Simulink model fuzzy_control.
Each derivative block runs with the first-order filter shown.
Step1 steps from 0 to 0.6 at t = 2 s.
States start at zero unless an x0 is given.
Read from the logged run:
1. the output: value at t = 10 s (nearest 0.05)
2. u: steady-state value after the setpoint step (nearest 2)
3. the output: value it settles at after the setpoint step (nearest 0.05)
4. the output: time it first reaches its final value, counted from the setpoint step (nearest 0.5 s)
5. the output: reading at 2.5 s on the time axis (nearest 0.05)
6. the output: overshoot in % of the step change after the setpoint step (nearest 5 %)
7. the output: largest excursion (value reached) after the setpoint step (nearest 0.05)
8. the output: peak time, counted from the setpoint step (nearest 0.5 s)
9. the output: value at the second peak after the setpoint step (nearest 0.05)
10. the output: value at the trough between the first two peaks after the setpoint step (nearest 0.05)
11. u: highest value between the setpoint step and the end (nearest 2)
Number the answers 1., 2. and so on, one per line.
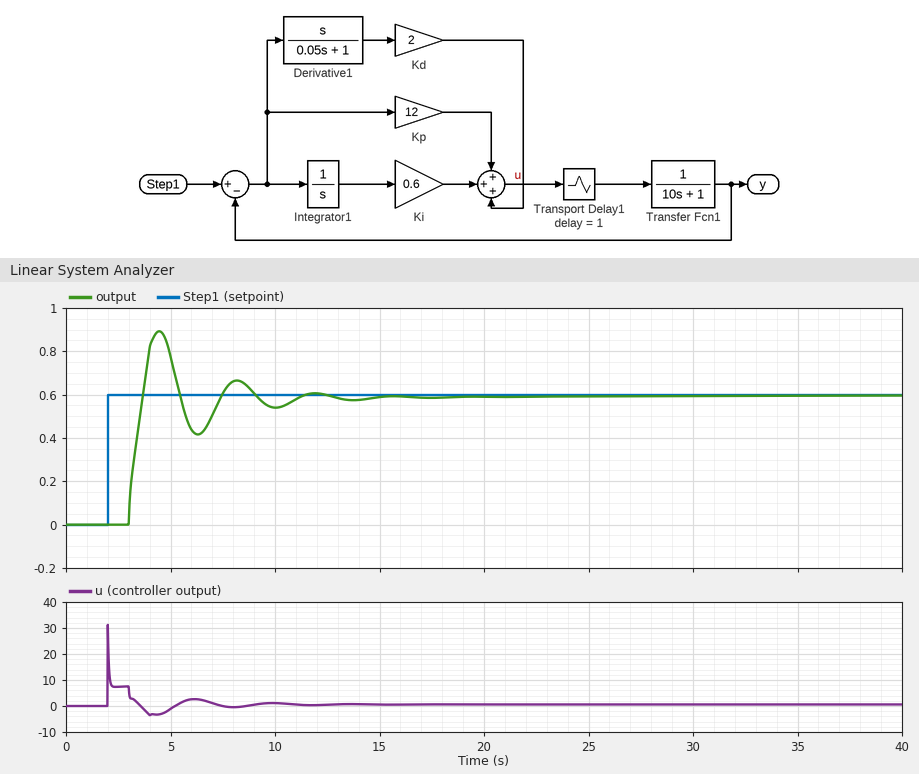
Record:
1. 0.55
2. 0
3. 0.60
4. 1.5 s
5. 0.00
6. 50 %
7. 0.90
8. 2.5 s
9. 0.65
10. 0.40
11. 32
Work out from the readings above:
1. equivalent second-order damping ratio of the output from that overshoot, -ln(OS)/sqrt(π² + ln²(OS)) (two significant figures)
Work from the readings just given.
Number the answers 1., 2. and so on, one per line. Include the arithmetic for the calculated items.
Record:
1. ln(0.5) = -0.693; 0.693 / sqrt(9.870 + 0.480) = 0.22
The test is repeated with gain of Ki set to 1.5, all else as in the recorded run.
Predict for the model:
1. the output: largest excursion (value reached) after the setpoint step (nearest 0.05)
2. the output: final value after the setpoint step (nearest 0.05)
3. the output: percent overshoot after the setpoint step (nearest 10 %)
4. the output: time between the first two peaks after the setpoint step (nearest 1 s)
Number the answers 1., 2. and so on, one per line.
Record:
1. 0.95
2. 0.60
3. 60 %
4. 4 s
